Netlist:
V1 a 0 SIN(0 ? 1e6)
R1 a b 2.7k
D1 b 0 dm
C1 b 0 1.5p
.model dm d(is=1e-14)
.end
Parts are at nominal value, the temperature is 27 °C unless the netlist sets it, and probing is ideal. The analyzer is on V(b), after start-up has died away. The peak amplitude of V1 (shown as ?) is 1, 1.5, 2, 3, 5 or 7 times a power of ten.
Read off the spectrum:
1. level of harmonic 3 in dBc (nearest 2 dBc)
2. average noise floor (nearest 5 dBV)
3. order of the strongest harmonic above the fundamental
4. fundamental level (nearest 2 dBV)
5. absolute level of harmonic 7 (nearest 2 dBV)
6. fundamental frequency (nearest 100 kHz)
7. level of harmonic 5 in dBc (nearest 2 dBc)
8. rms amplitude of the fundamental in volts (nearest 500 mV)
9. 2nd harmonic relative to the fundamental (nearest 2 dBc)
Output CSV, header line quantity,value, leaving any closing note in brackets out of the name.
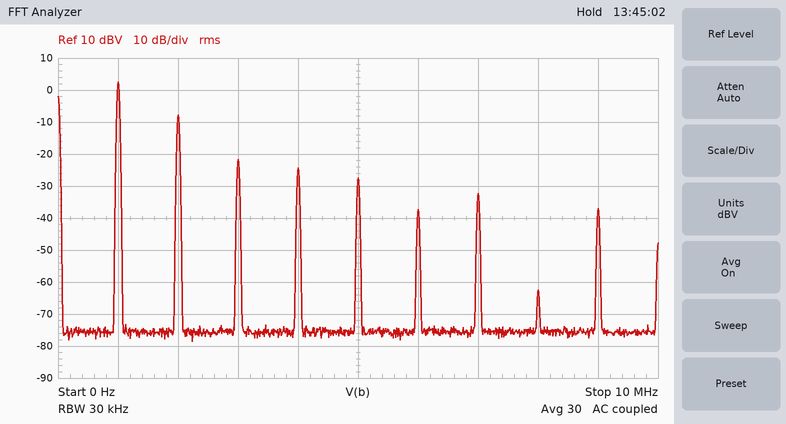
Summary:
quantity,value
level of harmonic 3 in dBc,-24 dBc
average noise floor,-75 dBV
order of the strongest harmonic above the fundamental,2
fundamental level,2 dBV
absolute level of harmonic 7,-32 dBV
fundamental frequency,1.0 MHz
level of harmonic 5 in dBc,-30 dBc
rms amplitude of the fundamental in volts,1.5 V
2nd harmonic relative to the fundamental,-10 dBc
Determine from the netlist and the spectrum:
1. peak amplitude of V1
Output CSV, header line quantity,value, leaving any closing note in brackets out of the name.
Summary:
quantity,value
peak amplitude of V1,3 V
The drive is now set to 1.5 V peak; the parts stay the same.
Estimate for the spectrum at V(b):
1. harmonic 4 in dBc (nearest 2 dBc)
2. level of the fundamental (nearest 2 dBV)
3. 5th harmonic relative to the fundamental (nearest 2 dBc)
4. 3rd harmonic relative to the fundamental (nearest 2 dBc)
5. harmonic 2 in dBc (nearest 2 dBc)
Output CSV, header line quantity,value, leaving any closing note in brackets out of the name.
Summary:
quantity,value
harmonic 4 in dBc,-48 dBc
level of the fundamental,-2 dBV
5th harmonic relative to the fundamental,-32 dBc
3rd harmonic relative to the fundamental,-22 dBc
harmonic 2 in dBc,-14 dBc
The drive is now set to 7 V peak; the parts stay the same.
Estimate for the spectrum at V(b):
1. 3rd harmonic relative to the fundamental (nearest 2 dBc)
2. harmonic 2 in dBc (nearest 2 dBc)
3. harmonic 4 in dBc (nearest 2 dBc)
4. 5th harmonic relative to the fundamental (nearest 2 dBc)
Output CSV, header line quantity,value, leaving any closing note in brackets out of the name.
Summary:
quantity,value
3rd harmonic relative to the fundamental,-30 dBc
harmonic 2 in dBc,-8 dBc
harmonic 4 in dBc,-24 dBc
5th harmonic relative to the fundamental,-34 dBc
